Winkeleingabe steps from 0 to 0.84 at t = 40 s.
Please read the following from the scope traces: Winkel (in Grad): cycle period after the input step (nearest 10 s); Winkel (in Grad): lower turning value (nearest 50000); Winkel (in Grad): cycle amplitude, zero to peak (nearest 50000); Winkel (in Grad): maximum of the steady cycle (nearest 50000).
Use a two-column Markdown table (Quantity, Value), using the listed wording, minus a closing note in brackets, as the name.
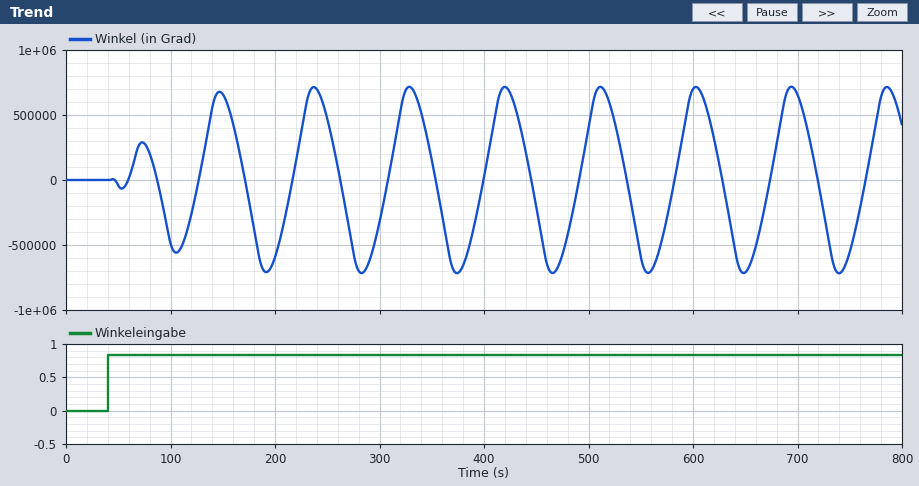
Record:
| Quantity | Value |
|---|---|
| Winkel (in Grad): cycle period after the input step | 90 s |
| Winkel (in Grad): lower turning value | -700000 |
| Winkel (in Grad): cycle amplitude, zero to peak | 700000 |
| Winkel (in Grad): maximum of the steady cycle | 700000 |
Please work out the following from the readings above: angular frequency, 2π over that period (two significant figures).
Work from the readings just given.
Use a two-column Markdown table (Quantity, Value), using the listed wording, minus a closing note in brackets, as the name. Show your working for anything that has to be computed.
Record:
| Quantity | Value |
|---|---|
| angular frequency, 2π over that period | 2π / 90 = 0.070 rad/s |
